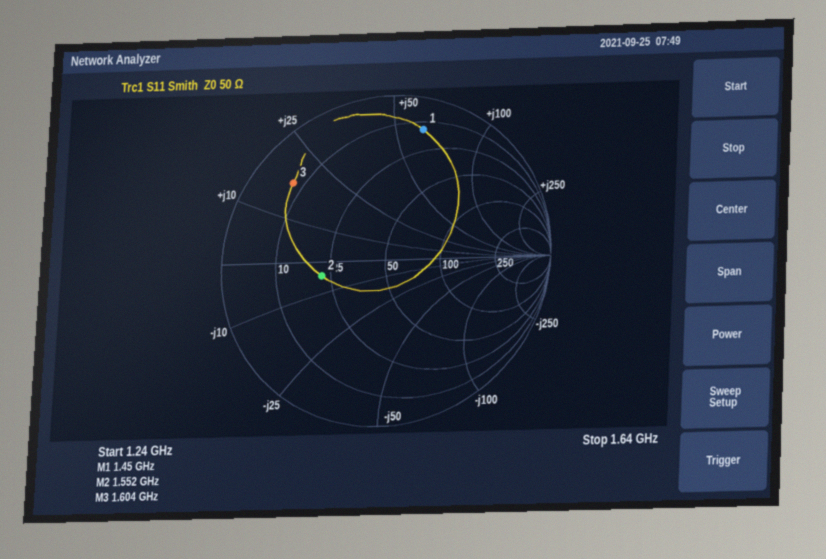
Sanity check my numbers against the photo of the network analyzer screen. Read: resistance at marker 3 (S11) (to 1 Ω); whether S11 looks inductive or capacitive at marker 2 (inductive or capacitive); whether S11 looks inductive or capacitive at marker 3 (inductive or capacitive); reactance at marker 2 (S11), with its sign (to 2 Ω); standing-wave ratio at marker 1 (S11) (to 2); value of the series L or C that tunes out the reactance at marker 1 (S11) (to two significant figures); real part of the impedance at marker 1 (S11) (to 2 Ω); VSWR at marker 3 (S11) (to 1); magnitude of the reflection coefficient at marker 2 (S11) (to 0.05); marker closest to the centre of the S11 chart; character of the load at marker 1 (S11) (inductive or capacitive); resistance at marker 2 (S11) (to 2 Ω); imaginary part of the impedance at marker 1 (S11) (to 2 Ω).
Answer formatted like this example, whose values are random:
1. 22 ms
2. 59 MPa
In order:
1. 8 Ω
2. capacitive
3. inductive
4. -4 Ω
5. 10
6. 1.8 pF
7. 14 Ω
8. 7
9. 0.40
10. marker 2
11. inductive
12. 22 Ω
13. +62 Ω
